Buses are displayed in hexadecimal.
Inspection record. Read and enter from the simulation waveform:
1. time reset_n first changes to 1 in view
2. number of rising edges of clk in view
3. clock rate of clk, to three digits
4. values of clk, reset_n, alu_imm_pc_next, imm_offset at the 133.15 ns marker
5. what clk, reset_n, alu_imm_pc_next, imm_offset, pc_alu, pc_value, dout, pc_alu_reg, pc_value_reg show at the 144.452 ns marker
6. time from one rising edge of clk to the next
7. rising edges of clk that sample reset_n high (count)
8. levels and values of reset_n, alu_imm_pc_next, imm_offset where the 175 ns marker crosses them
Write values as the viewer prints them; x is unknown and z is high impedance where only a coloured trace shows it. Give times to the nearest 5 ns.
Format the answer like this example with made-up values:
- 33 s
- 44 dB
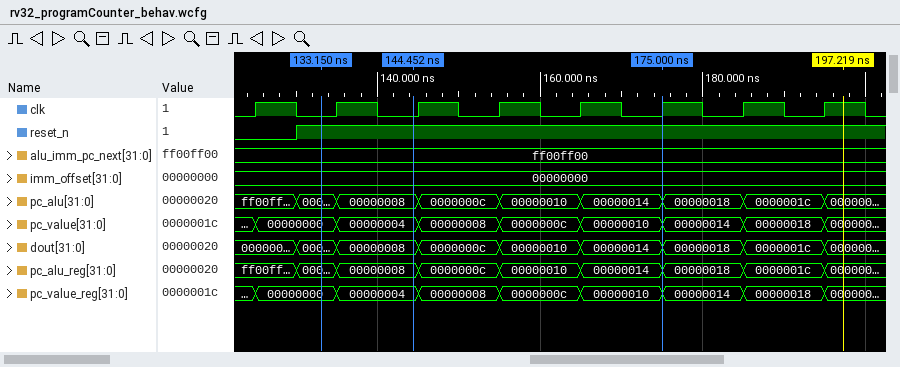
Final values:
- 130 ns
- 8
- 100 MHz
- clk=0, reset_n=1, alu_imm_pc_next=ff00ff00, imm_offset=00000000
- clk=0, reset_n=1, alu_imm_pc_next=ff00ff00, imm_offset=00000000, pc_alu=00000008, pc_value=00000004, dout=00000008, pc_alu_reg=00000008, pc_value_reg=00000004
- 10 ns
- 7
- reset_n=1, alu_imm_pc_next=ff00ff00, imm_offset=00000000
